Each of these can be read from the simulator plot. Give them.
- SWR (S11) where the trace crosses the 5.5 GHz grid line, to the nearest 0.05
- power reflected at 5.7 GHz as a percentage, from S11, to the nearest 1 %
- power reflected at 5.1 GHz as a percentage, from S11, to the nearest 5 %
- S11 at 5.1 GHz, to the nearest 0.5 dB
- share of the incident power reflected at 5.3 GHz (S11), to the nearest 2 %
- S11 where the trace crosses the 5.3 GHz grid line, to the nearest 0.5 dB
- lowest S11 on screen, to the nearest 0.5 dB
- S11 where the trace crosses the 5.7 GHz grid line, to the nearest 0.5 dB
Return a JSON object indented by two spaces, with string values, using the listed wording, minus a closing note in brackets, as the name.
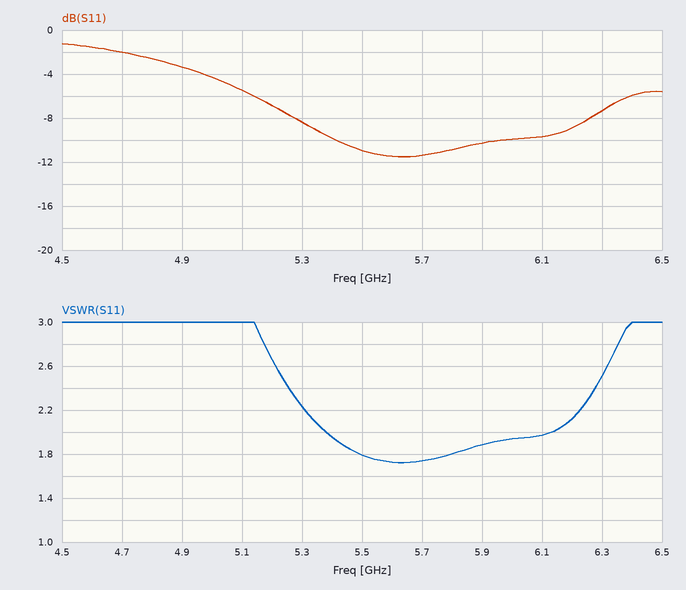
{
  "SWR (S11) where the trace crosses the 5.5 GHz grid line, to the nearest 0.05": "1.80",
  "power reflected at 5.7 GHz as a percentage, from S11, to the nearest 1 %": "7 %",
  "power reflected at 5.1 GHz as a percentage, from S11, to the nearest 5 %": "30 %",
  "S11 at 5.1 GHz, to the nearest 0.5 dB": "-5.5 dB",
  "share of the incident power reflected at 5.3 GHz (S11), to the nearest 2 %": "14 %",
  "S11 where the trace crosses the 5.3 GHz grid line, to the nearest 0.5 dB": "-8.5 dB",
  "lowest S11 on screen, to the nearest 0.5 dB": "-11.5 dB",
  "S11 where the trace crosses the 5.7 GHz grid line, to the nearest 0.5 dB": "-11.5 dB"
}
